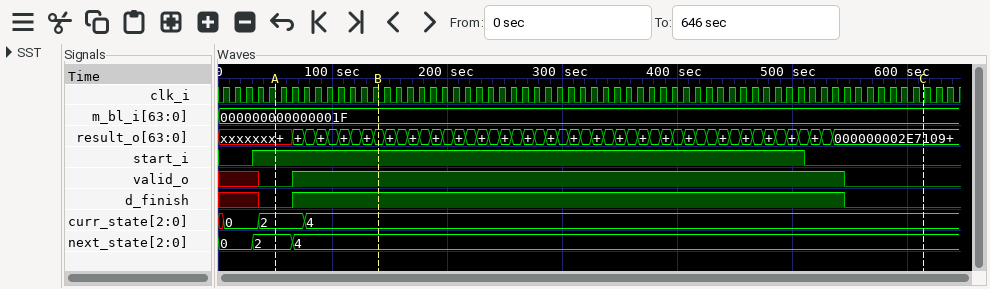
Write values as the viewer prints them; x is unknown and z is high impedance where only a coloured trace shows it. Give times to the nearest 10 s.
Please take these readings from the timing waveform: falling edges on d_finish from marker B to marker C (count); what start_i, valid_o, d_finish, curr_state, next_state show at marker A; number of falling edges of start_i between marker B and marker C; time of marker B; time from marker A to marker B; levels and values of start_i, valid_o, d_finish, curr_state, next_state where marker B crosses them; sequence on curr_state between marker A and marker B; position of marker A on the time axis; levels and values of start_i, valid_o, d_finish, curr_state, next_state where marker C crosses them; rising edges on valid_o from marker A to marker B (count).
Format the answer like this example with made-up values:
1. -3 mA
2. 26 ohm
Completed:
1. 1
2. start_i=1, valid_o=0, d_finish=0, curr_state=2, next_state=2
3. 1
4. 140 s
5. 90 s
6. start_i=1, valid_o=1, d_finish=1, curr_state=4, next_state=4
7. 2, 4
8. 50 s
9. start_i=0, valid_o=0, d_finish=0, curr_state=4, next_state=4
10. 1
